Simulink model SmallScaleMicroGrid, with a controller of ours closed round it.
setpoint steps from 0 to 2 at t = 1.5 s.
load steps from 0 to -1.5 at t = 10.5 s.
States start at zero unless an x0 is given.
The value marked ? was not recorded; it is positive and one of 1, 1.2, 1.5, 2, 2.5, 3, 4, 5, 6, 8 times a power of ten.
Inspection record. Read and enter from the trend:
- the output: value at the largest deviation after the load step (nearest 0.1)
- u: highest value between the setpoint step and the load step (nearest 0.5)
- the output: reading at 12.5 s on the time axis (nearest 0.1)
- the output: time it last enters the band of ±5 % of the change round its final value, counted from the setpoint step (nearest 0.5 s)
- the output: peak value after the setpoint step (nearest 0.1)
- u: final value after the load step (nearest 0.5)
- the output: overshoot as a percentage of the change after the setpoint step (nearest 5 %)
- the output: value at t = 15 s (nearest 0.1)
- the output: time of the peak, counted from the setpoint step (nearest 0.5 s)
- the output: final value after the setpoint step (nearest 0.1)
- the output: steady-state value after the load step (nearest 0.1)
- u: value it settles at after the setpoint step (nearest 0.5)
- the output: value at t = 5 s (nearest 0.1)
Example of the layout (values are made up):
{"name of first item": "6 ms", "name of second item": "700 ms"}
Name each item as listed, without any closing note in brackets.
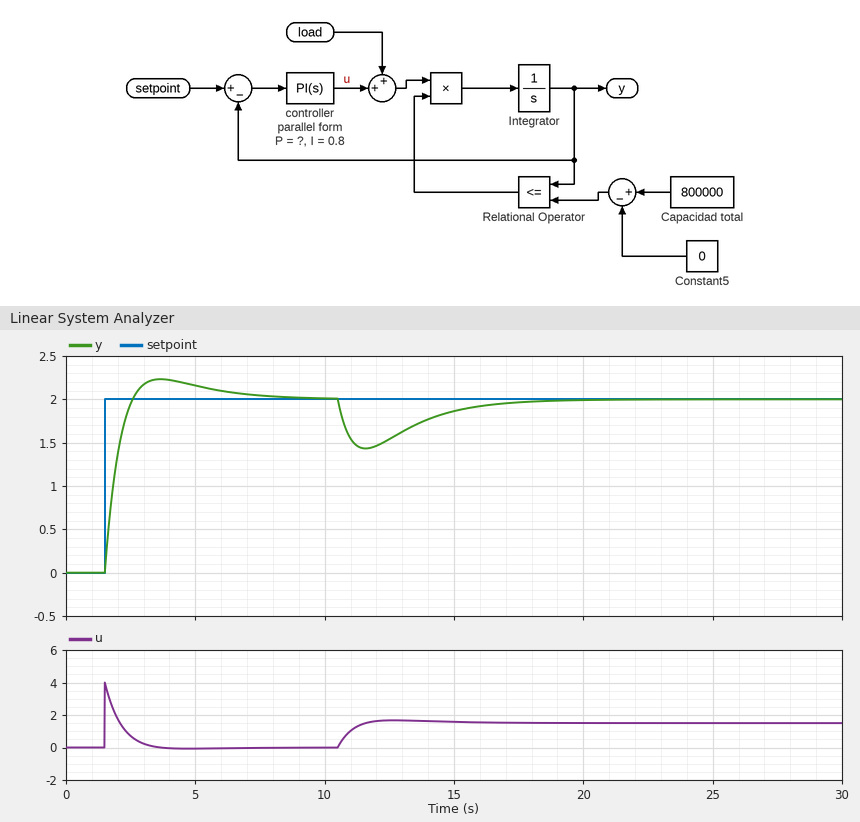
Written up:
{"the output: value at the largest deviation after the load step": "1.4", "u: highest value between the setpoint step and the load step": "4.0", "the output: reading at 12.5 s on the time axis": "1.5", "the output: time it last enters the band of ±5 % of the change round its final value, counted from the setpoint step": "4.5 s", "the output: peak value after the setpoint step": "2.2", "u: final value after the load step": "1.5", "the output: overshoot as a percentage of the change after the setpoint step": "10 %", "the output: value at t = 15 s": "1.9", "the output: time of the peak, counted from the setpoint step": "2.0 s", "the output: final value after the setpoint step": "2.0", "the output: steady-state value after the load step": "2.0", "u: value it settles at after the setpoint step": "0.0", "the output: value at t = 5 s": "2.2"}
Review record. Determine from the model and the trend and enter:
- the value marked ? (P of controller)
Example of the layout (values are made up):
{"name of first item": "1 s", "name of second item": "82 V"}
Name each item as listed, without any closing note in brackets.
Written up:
{"the value marked ?": "2"}
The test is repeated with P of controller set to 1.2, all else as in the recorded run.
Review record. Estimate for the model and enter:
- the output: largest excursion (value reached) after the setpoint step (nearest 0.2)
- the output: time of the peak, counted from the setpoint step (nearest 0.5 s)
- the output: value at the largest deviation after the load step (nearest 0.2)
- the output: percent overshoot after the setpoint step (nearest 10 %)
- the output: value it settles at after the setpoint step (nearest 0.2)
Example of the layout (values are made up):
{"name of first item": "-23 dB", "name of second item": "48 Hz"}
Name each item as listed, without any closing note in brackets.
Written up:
{"the output: largest excursion (value reached) after the setpoint step": "2.4", "the output: time of the peak, counted from the setpoint step": "2.5 s", "the output: value at the largest deviation after the load step": "1.2", "the output: percent overshoot after the setpoint step": "20 %", "the output: value it settles at after the setpoint step": "2.0"}
